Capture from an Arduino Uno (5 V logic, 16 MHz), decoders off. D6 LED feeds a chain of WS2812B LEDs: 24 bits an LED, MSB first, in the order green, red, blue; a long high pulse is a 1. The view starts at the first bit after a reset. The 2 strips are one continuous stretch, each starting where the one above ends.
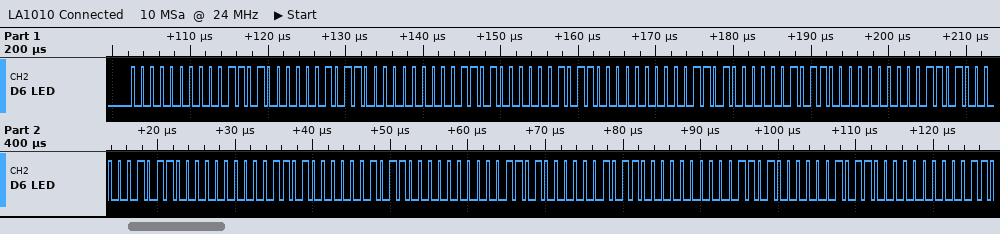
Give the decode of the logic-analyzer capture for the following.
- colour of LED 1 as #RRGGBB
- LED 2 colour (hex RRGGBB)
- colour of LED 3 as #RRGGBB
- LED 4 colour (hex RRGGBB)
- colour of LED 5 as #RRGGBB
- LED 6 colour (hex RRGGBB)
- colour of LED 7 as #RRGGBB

#34000B
#34000B
#34000B
#34000B
#34000B
#34000B
#34000B
